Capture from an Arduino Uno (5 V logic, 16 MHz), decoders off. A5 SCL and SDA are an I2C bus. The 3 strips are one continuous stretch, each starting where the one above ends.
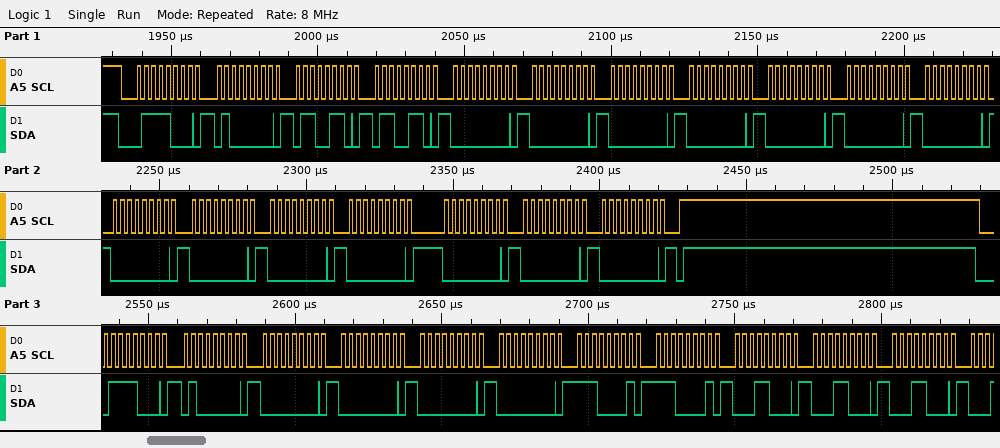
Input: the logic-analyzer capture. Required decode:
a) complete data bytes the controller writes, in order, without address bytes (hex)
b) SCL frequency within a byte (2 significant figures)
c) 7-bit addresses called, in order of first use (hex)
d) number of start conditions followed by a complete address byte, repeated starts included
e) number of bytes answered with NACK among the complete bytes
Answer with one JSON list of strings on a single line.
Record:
["40 66 66 00 00 00 00 00 00 00 00 00 00 00 00 00 00 40 00 00 00 00 E1 E1 18 18 18", "400 kHz", "0x3C", "2", "0"]
